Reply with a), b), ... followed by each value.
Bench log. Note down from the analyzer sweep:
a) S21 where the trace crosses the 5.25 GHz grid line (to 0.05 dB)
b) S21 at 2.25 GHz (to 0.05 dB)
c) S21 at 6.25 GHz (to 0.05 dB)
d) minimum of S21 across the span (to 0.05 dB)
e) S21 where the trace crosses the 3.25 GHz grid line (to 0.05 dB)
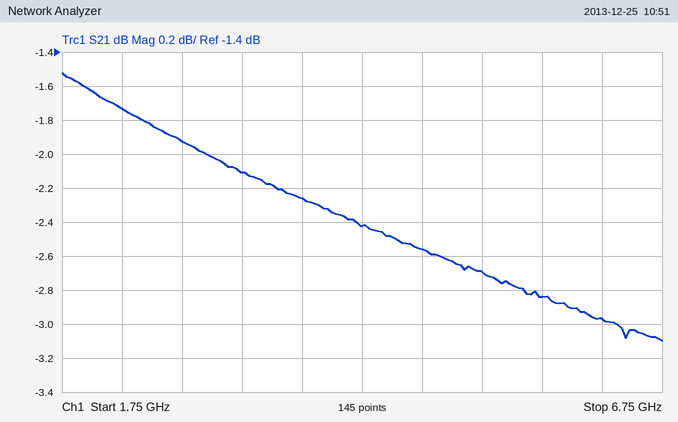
a) -2.70 dB
b) -1.75 dB
c) -2.95 dB
d) -3.10 dB
e) -2.10 dB
